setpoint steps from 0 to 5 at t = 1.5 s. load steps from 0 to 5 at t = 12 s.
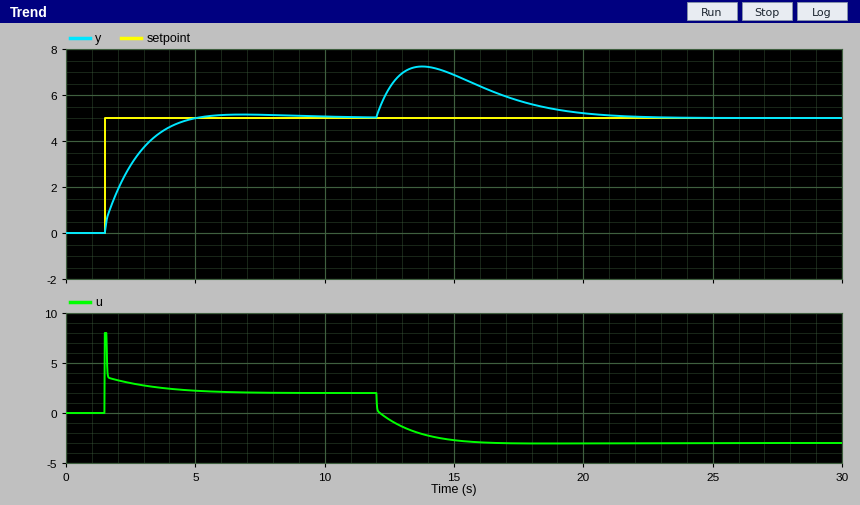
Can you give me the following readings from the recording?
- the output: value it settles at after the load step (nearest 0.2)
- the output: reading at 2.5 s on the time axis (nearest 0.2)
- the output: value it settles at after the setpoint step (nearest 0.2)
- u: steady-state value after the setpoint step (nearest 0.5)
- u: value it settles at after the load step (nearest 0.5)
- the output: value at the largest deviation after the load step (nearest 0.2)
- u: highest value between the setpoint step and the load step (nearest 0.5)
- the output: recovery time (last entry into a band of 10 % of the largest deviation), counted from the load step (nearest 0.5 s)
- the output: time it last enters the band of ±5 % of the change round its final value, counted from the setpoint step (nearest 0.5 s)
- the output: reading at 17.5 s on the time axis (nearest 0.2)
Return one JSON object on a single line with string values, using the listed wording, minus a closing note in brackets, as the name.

{"the output: value it settles at after the load step": "5.0", "the output: reading at 2.5 s on the time axis": "3.0", "the output: value it settles at after the setpoint step": "5.0", "u: steady-state value after the setpoint step": "2.0", "u: value it settles at after the load step": "-3.0", "the output: value at the largest deviation after the load step": "7.2", "u: highest value between the setpoint step and the load step": "8.0", "the output: recovery time (last entry into a band of 10 % of the largest deviation), counted from the load step": "8.0 s", "the output: time it last enters the band of ±5 % of the change round its final value, counted from the setpoint step": "3.0 s", "the output: reading at 17.5 s on the time axis": "5.8"}
